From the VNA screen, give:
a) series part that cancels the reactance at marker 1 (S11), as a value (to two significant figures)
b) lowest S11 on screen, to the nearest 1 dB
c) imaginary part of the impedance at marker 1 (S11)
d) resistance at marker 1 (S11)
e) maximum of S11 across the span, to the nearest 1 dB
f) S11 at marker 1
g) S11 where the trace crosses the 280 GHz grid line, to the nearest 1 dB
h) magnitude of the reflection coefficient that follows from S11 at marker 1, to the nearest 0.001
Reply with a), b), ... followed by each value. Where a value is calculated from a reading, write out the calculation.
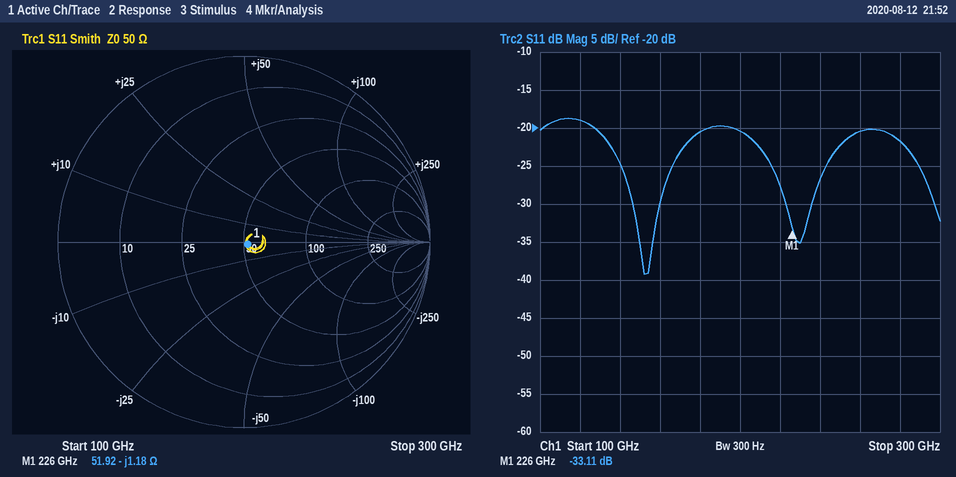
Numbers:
a) L = 1.18 Ω/(2π × 226 GHz) ≈ 831 fH, so 830 fH to two significant figures
b) -39 dB
c) -1.18 Ω
d) 51.92 Ω
e) -19 dB
f) -33.11 dB
g) -22 dB
h) 10^(-33.11/20) ≈ 0.022
